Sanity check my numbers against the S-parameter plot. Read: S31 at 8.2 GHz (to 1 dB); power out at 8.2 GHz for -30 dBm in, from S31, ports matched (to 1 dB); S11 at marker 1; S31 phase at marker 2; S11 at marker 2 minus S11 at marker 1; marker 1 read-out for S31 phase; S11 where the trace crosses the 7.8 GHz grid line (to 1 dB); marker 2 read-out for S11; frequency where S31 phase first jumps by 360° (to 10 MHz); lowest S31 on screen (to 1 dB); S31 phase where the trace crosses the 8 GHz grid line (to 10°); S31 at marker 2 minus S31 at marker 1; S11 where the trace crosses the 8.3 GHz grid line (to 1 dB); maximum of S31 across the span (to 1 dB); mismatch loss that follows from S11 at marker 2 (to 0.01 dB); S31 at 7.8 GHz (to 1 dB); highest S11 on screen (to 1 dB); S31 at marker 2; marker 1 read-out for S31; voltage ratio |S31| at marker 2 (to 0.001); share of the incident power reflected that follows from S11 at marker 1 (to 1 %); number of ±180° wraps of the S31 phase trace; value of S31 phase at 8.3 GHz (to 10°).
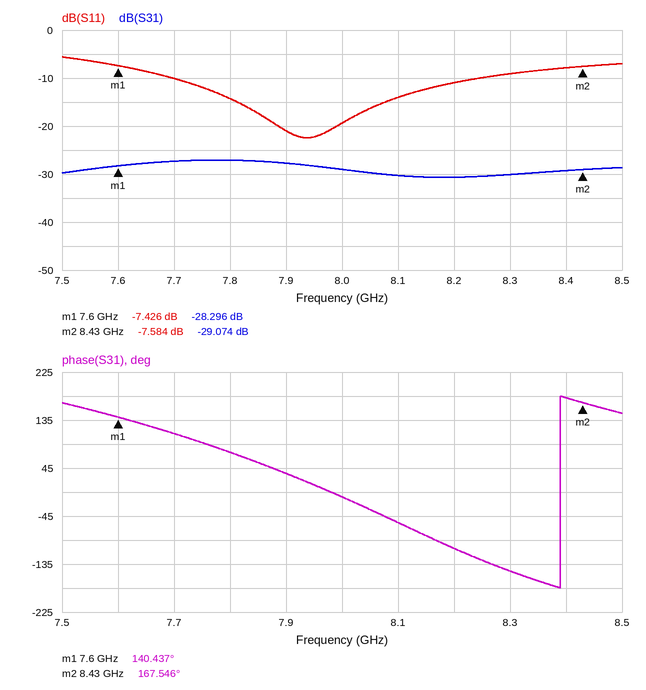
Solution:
-31 dB
-61 dBm
-7.426 dB
167.546°
-0.158 dB
140.437°
-14 dB
-7.584 dB
8.39 GHz
-31 dB
-10°
-0.778 dB
-9 dB
-27 dB
0.83 dB
-27 dB
-6 dB
-29.074 dB
-28.296 dB
0.035
18 %
1
-150°
